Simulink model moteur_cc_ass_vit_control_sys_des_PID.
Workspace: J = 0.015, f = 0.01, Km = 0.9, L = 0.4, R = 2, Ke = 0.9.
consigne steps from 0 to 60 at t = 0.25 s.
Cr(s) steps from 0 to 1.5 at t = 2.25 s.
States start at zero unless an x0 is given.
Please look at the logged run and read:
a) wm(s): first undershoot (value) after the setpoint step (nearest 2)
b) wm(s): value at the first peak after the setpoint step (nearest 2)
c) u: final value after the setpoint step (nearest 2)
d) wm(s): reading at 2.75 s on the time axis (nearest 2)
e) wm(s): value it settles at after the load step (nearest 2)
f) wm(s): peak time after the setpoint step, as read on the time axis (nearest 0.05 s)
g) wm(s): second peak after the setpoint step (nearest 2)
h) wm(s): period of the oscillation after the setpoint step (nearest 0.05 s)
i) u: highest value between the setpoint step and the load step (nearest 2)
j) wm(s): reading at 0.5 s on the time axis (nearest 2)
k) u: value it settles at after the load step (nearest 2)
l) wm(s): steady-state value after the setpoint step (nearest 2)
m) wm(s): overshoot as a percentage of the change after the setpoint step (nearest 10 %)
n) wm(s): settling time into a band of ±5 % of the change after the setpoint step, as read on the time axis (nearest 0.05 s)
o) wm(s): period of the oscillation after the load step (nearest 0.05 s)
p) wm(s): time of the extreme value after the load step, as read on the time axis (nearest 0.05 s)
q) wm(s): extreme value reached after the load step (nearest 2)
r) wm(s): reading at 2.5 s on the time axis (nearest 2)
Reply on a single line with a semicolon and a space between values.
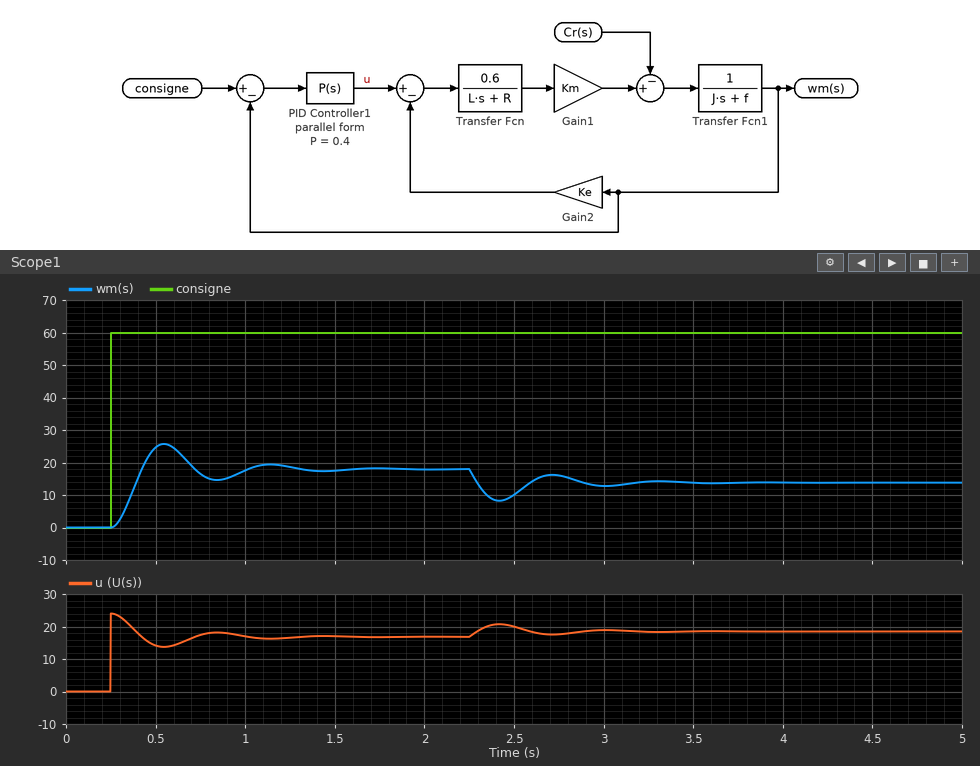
14; 26; 16; 16; 14; 0.55 s; 20; 0.60 s; 24; 24; 18; 18; 40 %; 1.25 s; 0.60 s; 2.40 s; 8; 10
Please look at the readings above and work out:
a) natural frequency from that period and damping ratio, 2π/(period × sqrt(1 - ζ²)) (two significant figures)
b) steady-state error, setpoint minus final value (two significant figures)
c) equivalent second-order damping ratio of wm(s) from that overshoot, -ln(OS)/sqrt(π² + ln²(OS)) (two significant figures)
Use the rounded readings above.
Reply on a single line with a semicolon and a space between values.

11 rad/s; 42; 0.28
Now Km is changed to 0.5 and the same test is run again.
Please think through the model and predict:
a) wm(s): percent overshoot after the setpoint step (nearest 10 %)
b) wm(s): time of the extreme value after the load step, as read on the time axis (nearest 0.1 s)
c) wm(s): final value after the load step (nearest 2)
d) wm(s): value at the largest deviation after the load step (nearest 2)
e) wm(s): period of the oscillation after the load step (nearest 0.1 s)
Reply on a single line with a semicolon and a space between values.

30 %; 2.5 s; 10; 4; 0.8 s
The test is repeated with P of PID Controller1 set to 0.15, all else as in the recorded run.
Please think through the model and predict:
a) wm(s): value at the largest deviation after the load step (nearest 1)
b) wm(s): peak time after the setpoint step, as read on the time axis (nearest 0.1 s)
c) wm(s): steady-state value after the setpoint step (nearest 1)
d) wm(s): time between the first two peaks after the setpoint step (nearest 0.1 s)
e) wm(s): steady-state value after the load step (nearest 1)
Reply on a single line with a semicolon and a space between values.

-3; 0.6 s; 8; 0.7 s; 3
